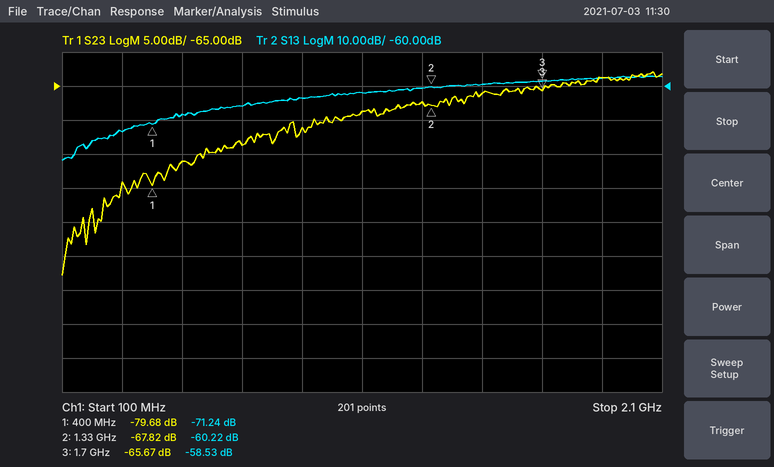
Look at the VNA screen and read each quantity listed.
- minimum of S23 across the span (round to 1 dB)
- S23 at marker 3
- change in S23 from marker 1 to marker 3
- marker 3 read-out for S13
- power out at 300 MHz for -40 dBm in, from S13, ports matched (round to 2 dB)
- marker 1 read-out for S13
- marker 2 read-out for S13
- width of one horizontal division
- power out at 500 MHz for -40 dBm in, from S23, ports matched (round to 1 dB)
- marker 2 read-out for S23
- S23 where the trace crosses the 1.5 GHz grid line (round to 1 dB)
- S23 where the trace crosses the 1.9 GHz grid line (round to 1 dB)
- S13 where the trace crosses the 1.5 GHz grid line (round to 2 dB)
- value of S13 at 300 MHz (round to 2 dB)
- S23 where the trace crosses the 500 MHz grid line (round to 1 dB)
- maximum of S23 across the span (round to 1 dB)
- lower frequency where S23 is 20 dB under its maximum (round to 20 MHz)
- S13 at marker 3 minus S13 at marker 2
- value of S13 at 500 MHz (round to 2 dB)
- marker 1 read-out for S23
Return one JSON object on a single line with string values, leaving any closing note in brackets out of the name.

{"minimum of S23 across the span": "-93 dB", "S23 at marker 3": "-65.67 dB", "change in S23 from marker 1 to marker 3": "14.01 dB", "marker 3 read-out for S13": "-58.53 dB", "power out at 300 MHz for -40 dBm in, from S13, ports matched": "-114 dBm", "marker 1 read-out for S13": "-71.24 dB", "marker 2 read-out for S13": "-60.22 dB", "width of one horizontal division": "200 MHz", "power out at 500 MHz for -40 dBm in, from S23, ports matched": "-116 dBm", "marker 2 read-out for S23": "-67.82 dB", "S23 where the trace crosses the 1.5 GHz grid line": "-66 dB", "S23 where the trace crosses the 1.9 GHz grid line": "-64 dB", "S13 where the trace crosses the 1.5 GHz grid line": "-60 dB", "value of S13 at 300 MHz": "-74 dB", "S23 where the trace crosses the 500 MHz grid line": "-76 dB", "maximum of S23 across the span": "-63 dB", "lower frequency where S23 is 20 dB under its maximum": "240 MHz", "S13 at marker 3 minus S13 at marker 2": "1.69 dB", "value of S13 at 500 MHz": "-68 dB", "marker 1 read-out for S23": "-79.68 dB"}
